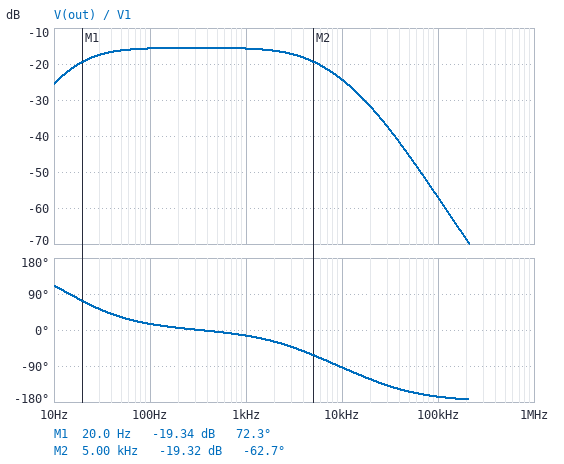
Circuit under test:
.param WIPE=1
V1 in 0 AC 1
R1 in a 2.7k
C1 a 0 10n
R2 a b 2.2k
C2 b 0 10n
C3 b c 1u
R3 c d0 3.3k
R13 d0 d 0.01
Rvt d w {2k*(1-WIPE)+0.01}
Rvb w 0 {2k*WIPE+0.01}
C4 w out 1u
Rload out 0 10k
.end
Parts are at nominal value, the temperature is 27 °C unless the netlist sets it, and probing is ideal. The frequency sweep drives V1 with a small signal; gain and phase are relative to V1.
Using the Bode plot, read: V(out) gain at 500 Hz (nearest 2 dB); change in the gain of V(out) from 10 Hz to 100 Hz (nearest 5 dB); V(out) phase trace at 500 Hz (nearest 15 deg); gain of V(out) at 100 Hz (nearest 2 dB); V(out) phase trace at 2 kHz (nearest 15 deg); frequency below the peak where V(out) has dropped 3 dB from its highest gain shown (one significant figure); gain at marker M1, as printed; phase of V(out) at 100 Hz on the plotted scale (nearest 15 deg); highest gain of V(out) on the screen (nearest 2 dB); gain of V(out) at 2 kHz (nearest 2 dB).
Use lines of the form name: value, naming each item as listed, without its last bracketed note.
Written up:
V(out) gain at 500 Hz: -16 dB
change in the gain of V(out) from 10 Hz to 100 Hz: 10 dB
V(out) phase trace at 500 Hz: 0 deg
gain of V(out) at 100 Hz: -16 dB
V(out) phase trace at 2 kHz: -30 deg
frequency below the peak where V(out) has dropped 3 dB from its highest gain shown: 20 Hz
gain at marker M1, as printed: -19.34 dB
phase of V(out) at 100 Hz on the plotted scale: 15 deg
highest gain of V(out) on the screen: -16 dB
gain of V(out) at 2 kHz: -16 dB
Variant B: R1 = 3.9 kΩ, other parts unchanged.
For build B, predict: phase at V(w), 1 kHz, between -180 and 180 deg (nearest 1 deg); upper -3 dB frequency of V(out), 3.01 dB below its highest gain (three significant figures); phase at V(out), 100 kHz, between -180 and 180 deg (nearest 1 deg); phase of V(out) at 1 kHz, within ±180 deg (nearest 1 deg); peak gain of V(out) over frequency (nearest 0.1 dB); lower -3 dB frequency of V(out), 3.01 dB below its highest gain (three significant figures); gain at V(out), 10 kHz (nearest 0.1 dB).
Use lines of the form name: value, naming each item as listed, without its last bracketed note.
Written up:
phase at V(w), 1 kHz, between -180 and 180 deg: -18 deg
upper -3 dB frequency of V(out), 3.01 dB below its highest gain: 3.55 kHz
phase at V(out), 100 kHz, between -180 and 180 deg: -168 deg
phase of V(out) at 1 kHz, within ±180 deg: -17 deg
peak gain of V(out) over frequency: -16.5 dB
lower -3 dB frequency of V(out), 3.01 dB below its highest gain: 21.7 Hz
gain at V(out), 10 kHz: -26.9 dB
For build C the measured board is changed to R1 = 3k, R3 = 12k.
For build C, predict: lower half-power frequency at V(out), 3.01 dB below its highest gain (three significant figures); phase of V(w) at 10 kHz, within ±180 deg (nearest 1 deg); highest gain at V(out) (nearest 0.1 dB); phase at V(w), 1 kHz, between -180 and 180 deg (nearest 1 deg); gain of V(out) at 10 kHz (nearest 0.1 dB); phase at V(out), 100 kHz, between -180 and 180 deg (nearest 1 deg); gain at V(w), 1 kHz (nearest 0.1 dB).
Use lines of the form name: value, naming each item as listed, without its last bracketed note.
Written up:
lower half-power frequency at V(out), 3.01 dB below its highest gain: 17.1 Hz
phase of V(w) at 10 kHz, within ±180 deg: -103 deg
highest gain at V(out): -21.1 dB
phase at V(w), 1 kHz, between -180 and 180 deg: -22 deg
gain of V(out) at 10 kHz: -33.2 dB
phase at V(out), 100 kHz, between -180 and 180 deg: -168 deg
gain at V(w), 1 kHz: -21.6 dB
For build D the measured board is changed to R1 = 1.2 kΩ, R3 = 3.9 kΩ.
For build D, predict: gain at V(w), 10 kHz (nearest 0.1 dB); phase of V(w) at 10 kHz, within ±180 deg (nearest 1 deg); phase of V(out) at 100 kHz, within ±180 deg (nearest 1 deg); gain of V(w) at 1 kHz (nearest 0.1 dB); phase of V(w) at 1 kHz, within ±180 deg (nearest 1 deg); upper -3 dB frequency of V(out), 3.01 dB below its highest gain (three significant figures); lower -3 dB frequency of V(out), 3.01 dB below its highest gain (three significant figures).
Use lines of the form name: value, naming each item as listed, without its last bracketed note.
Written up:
gain at V(w), 10 kHz: -20.7 dB
phase of V(w) at 10 kHz, within ±180 deg: -80 deg
phase of V(out) at 100 kHz, within ±180 deg: -163 deg
gain of V(w) at 1 kHz: -14.7 dB
phase of V(w) at 1 kHz, within ±180 deg: -10 deg
upper -3 dB frequency of V(out), 3.01 dB below its highest gain: 6.05 kHz
lower -3 dB frequency of V(out), 3.01 dB below its highest gain: 24.6 Hz
